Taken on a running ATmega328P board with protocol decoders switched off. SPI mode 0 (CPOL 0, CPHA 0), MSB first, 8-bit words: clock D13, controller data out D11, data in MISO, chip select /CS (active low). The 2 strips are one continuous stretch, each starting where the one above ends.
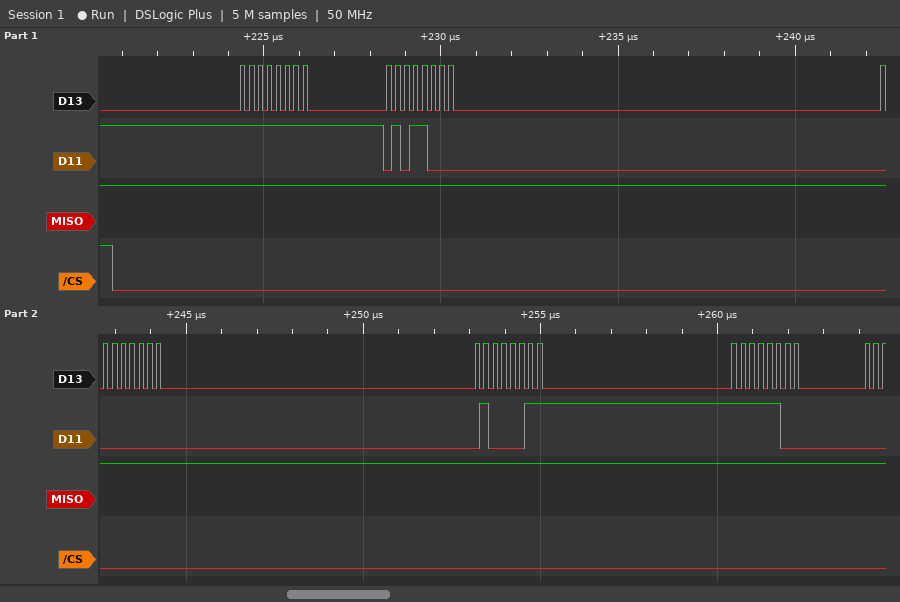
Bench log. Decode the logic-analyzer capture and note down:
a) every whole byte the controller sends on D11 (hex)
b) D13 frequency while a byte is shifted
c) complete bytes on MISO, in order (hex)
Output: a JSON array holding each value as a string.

["FF 58 00 43 FC", "4 MHz", "FF FF FF FF FF"]
